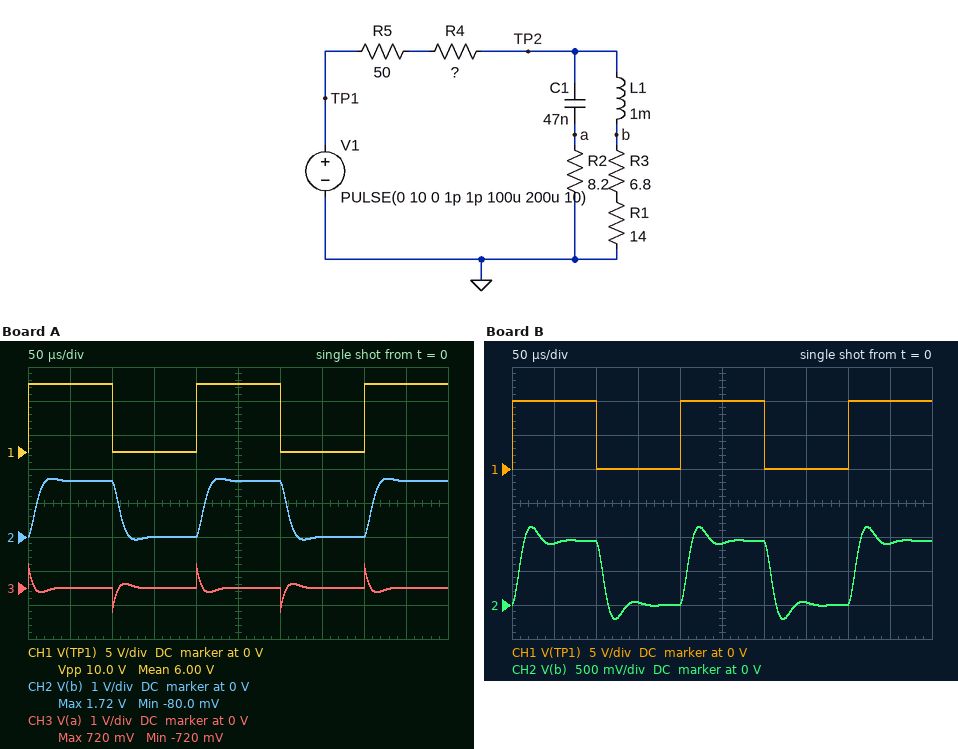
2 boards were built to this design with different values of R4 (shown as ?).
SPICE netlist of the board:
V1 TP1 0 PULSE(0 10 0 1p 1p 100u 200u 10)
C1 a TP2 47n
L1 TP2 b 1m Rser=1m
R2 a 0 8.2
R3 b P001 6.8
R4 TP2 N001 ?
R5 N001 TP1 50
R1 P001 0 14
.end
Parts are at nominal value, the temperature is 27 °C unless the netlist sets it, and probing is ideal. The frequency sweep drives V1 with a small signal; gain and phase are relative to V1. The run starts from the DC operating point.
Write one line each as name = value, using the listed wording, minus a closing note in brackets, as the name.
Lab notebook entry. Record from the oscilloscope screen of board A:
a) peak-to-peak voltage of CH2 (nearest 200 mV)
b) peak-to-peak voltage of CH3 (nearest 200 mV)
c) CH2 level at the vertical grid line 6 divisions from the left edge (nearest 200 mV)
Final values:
peak-to-peak voltage of CH2 = 1.8 V
peak-to-peak voltage of CH3 = 1.4 V
CH2 level at the vertical grid line 6 divisions from the left edge = 1.6 V
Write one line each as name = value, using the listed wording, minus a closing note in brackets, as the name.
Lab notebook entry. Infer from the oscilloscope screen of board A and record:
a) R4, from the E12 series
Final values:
R4, from the E12 series = 56 Ω
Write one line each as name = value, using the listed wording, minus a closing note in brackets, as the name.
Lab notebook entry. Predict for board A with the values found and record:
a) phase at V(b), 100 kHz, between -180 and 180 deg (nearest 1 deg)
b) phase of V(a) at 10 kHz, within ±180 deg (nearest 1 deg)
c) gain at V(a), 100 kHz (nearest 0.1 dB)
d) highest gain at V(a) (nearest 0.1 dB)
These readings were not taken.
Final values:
phase at V(b), 100 kHz, between -180 and 180 deg = -146 deg
phase of V(a) at 10 kHz, within ±180 deg = 127 deg
gain at V(a), 100 kHz = -22.9 dB
highest gain at V(a) = -22.9 dB
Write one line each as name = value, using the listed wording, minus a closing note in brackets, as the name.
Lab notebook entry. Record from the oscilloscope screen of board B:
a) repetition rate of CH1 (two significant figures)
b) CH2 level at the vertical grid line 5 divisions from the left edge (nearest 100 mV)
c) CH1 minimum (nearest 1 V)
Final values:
repetition rate of CH1 = 5.0 kHz
CH2 level at the vertical grid line 5 divisions from the left edge = 900 mV
CH1 minimum = 0 V
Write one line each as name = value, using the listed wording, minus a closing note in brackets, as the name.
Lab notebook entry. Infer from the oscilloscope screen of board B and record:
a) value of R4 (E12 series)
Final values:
value of R4 = 150 Ω
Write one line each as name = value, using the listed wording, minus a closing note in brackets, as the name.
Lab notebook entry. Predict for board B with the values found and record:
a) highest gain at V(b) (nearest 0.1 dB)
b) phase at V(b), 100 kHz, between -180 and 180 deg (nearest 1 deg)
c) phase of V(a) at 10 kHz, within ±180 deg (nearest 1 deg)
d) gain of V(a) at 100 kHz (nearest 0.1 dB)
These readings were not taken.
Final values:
highest gain at V(b) = -18.4 dB
phase at V(b), 100 kHz, between -180 and 180 deg = -154 deg
phase of V(a) at 10 kHz, within ±180 deg = 138 deg
gain of V(a) at 100 kHz = -27.8 dB
